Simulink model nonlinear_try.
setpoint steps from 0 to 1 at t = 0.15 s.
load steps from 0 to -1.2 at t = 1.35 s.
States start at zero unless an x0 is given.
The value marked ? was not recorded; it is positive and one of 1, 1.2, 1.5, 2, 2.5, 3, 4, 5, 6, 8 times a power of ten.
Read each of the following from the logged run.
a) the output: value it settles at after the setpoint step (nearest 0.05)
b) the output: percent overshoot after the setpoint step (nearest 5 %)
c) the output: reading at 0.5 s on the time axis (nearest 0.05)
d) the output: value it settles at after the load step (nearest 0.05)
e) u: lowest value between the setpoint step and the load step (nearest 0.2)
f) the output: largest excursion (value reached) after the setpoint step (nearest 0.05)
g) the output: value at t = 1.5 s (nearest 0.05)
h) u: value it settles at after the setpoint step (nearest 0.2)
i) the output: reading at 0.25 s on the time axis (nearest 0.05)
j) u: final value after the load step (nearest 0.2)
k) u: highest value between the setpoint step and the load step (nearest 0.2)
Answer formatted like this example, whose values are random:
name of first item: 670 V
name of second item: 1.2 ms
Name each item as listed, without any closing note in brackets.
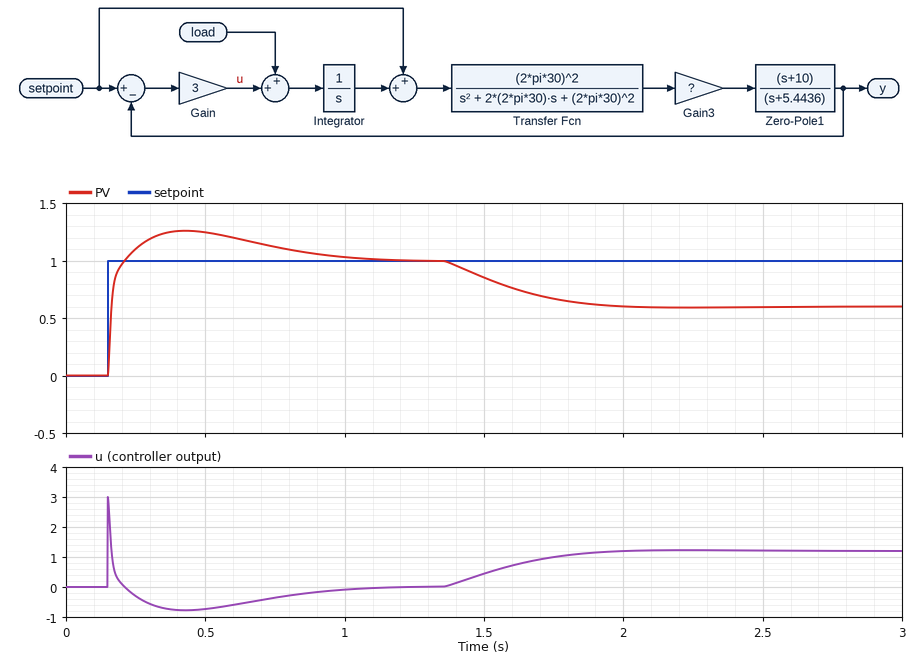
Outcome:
the output: value it settles at after the setpoint step: 1.00
the output: percent overshoot after the setpoint step: 25 %
the output: reading at 0.5 s on the time axis: 1.25
the output: value it settles at after the load step: 0.60
u: lowest value between the setpoint step and the load step: -0.8
the output: largest excursion (value reached) after the setpoint step: 1.25
the output: value at t = 1.5 s: 0.85
u: value it settles at after the setpoint step: 0.0
the output: reading at 0.25 s on the time axis: 1.10
u: final value after the load step: 1.2
u: highest value between the setpoint step and the load step: 3.0
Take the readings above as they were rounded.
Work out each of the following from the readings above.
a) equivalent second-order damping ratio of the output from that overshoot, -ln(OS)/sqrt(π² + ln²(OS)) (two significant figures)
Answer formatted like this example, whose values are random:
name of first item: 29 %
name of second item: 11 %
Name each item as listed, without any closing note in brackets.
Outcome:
equivalent second-order damping ratio of the output from that overshoot, -ln(OS)/sqrt(π² + ln²(OS)): 0.40
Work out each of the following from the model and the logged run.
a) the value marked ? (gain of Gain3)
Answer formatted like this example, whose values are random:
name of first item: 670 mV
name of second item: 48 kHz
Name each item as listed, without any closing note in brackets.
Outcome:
the value marked ?: 0.8
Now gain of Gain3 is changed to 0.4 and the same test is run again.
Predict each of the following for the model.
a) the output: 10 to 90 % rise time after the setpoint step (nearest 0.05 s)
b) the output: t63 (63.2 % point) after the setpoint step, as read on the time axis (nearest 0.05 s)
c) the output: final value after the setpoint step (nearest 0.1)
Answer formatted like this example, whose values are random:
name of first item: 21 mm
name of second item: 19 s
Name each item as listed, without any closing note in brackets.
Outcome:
the output: 10 to 90 % rise time after the setpoint step: 0.35 s
the output: t63 (63.2 % point) after the setpoint step, as read on the time axis: 0.25 s
the output: final value after the setpoint step: 1.0
